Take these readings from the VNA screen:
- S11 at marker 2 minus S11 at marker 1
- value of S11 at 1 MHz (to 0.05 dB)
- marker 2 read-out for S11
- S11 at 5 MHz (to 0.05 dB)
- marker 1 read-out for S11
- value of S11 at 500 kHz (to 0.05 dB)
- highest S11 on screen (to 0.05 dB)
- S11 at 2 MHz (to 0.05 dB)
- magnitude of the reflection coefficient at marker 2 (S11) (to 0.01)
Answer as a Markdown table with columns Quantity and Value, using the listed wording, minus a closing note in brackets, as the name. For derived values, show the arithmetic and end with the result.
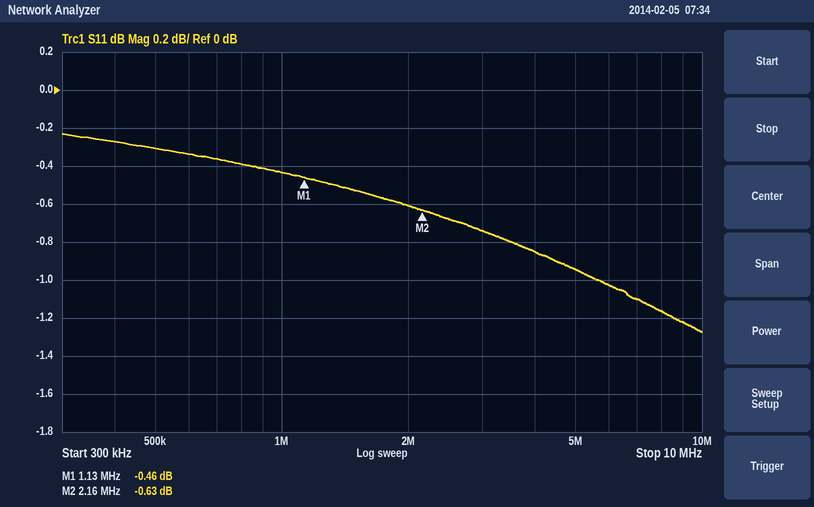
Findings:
| Quantity | Value |
|---|---|
| S11 at marker 2 minus S11 at marker 1 | -0.63 − (-0.46) = -0.17 dB |
| value of S11 at 1 MHz | -0.45 dB |
| marker 2 read-out for S11 | -0.63 dB |
| S11 at 5 MHz | -0.95 dB |
| marker 1 read-out for S11 | -0.46 dB |
| value of S11 at 500 kHz | -0.30 dB |
| highest S11 on screen | -0.25 dB |
| S11 at 2 MHz | -0.60 dB |
| magnitude of the reflection coefficient at marker 2 (S11) | 10^(-0.63/20) ≈ 0.93 |
